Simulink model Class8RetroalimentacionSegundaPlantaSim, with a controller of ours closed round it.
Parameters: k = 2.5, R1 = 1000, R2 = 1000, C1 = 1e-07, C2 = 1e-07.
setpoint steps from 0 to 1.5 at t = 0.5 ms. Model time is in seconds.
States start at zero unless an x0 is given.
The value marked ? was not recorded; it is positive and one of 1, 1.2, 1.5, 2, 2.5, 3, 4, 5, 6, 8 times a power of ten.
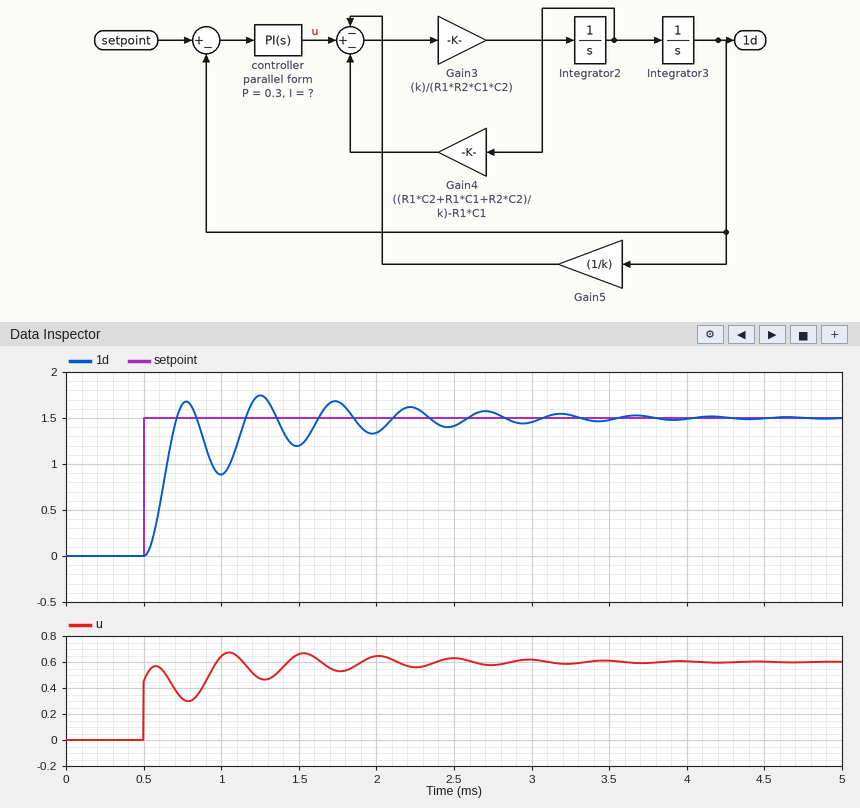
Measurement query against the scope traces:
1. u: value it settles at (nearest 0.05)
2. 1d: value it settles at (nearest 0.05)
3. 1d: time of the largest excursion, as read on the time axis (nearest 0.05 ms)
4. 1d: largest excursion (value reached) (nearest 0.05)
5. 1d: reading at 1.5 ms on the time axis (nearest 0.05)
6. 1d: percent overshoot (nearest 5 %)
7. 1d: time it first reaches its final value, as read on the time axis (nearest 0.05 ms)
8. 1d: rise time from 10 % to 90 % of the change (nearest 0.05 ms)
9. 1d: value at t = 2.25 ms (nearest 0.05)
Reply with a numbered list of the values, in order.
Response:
1. 0.60
2. 1.50
3. 1.25 ms
4. 1.75
5. 1.20
6. 15 %
7. 0.70 ms
8. 0.15 ms
9. 1.60
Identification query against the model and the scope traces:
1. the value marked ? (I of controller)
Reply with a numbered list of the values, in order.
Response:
1. 2000
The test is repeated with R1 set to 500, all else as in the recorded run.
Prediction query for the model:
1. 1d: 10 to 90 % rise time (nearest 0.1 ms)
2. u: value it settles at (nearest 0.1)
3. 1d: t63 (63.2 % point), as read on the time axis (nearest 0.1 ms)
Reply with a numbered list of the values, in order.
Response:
1. 0.5 ms
2. 0.6
3. 0.6 ms
